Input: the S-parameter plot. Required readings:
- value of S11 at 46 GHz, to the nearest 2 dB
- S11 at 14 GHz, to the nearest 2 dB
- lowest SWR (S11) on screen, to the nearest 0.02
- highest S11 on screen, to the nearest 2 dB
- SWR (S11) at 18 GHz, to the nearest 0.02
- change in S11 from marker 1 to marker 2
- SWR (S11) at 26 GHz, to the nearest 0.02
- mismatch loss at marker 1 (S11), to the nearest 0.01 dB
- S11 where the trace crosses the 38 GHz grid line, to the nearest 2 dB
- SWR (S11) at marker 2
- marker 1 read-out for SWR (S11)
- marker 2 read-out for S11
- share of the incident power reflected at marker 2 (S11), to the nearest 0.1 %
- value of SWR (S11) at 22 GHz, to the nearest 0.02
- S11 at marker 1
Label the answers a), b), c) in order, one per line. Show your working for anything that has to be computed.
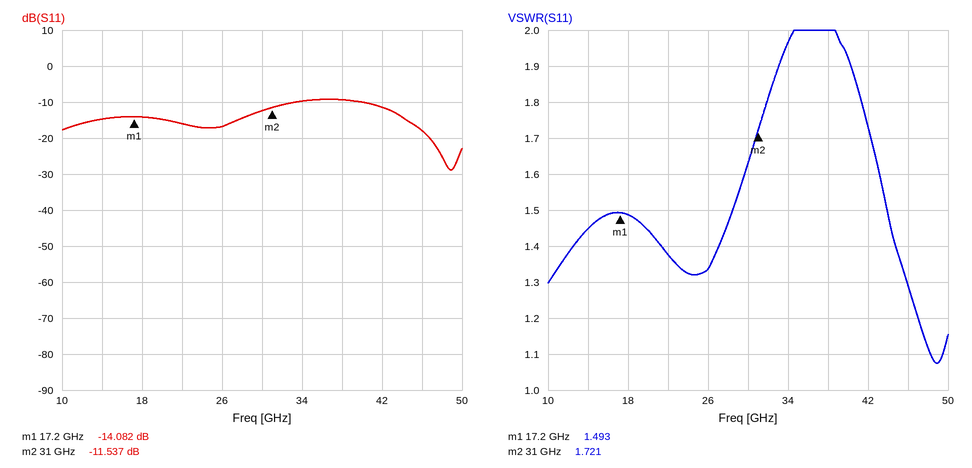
a) -18 dB
b) -14 dB
c) 1.08
d) -10 dB
e) 1.48
f) -11.537 − (-14.082) = 2.545 dB
g) 1.34
h) −10 log10(1 − 10^(-14.082/10)) ≈ 0.17 dB
i) -10 dB
j) 1.721
k) 1.493
l) -11.537 dB
m) 10^(-11.537/10) ≈ 7.0 %
n) 1.38
o) -14.082 dB
